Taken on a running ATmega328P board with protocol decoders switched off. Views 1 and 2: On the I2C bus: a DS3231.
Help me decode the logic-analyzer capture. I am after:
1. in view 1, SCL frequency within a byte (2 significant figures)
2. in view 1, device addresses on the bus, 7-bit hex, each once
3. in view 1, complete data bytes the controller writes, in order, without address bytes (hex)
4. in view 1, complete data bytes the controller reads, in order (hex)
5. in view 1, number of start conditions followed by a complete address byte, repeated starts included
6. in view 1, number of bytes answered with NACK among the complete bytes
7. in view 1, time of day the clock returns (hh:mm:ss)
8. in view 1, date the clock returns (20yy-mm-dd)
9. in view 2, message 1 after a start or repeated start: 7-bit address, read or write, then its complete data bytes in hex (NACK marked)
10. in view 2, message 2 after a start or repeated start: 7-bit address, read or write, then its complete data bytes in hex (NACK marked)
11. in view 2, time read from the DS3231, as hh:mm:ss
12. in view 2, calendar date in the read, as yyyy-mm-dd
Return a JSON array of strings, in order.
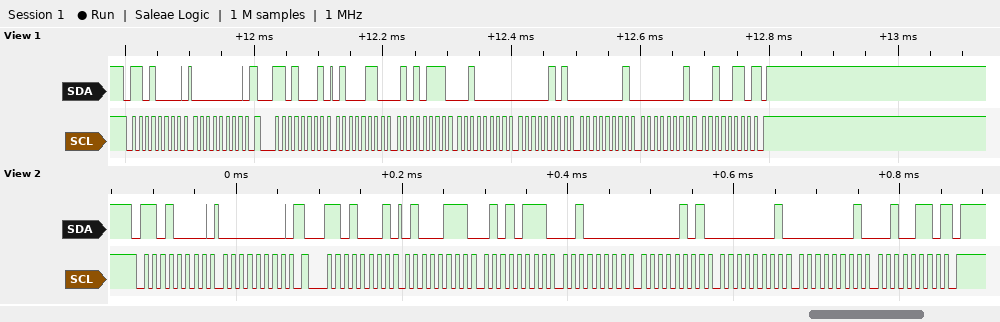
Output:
["100 kHz", "0x68", "00", "46 57 20 05 01 01 26", "2", "1", "20:57:46", "2026-01-01", "0x68 write: 00", "0x68 read: 47 57 20 05 01 01 26 NACK", "20:57:47", "2026-01-01"]
